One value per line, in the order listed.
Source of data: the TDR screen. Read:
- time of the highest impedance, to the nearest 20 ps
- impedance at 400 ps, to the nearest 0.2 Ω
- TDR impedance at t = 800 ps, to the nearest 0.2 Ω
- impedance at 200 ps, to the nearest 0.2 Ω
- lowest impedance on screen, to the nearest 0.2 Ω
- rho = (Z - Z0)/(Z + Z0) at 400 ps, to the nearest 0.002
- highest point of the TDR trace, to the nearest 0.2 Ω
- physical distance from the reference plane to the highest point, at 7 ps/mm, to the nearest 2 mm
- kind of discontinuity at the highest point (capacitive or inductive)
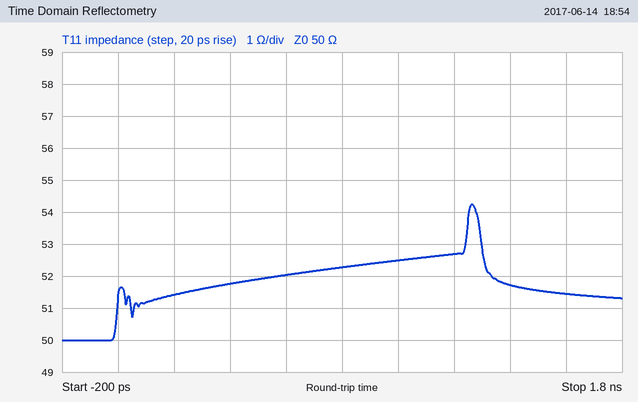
1.26 ns
51.8 Ω
52.2 Ω
51.4 Ω
50.0 Ω
+0.018
54.2 Ω
90 mm
inductive
